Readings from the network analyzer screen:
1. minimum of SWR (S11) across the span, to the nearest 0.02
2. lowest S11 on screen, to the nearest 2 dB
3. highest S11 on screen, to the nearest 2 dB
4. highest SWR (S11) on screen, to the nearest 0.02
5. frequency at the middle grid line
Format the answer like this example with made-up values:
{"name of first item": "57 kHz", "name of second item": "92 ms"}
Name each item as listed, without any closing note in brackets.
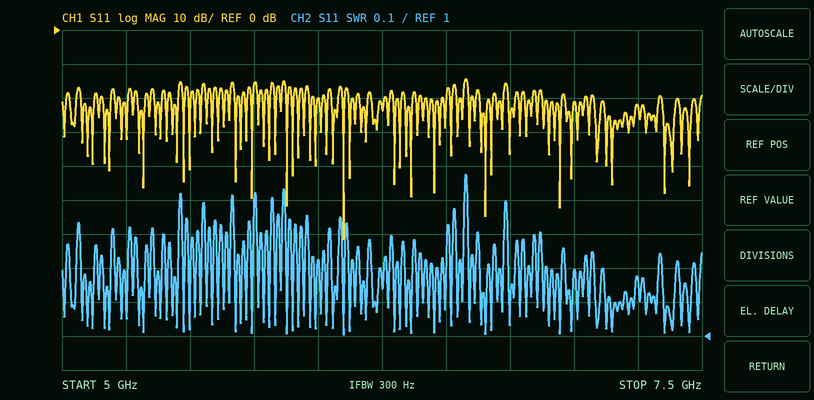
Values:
{"minimum of SWR (S11) across the span, to the nearest 0.02": "1.00", "lowest S11 on screen, to the nearest 2 dB": "-62 dB", "highest S11 on screen, to the nearest 2 dB": "-14 dB", "highest SWR (S11) on screen, to the nearest 0.02": "1.48", "frequency at the middle grid line": "6.25 GHz"}
